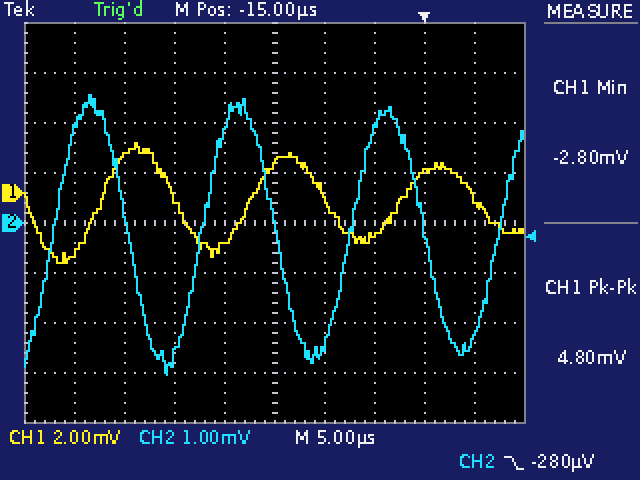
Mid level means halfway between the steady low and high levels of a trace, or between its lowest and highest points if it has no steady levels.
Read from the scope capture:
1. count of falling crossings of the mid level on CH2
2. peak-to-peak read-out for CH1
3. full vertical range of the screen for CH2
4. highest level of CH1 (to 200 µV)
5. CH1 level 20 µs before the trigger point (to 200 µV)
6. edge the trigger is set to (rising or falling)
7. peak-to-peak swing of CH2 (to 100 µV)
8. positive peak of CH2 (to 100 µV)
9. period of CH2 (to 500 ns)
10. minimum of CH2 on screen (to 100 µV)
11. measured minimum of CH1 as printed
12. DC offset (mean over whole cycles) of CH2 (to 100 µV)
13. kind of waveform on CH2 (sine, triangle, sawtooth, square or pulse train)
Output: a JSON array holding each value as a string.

["3", "4.80 mV", "8 mV", "2.0 mV", "-2.0 mV", "falling", "5.6 mV", "2.6 mV", "15.0 µs", "-3.0 mV", "-2.80 mV", "-200 µV", "sine"]
